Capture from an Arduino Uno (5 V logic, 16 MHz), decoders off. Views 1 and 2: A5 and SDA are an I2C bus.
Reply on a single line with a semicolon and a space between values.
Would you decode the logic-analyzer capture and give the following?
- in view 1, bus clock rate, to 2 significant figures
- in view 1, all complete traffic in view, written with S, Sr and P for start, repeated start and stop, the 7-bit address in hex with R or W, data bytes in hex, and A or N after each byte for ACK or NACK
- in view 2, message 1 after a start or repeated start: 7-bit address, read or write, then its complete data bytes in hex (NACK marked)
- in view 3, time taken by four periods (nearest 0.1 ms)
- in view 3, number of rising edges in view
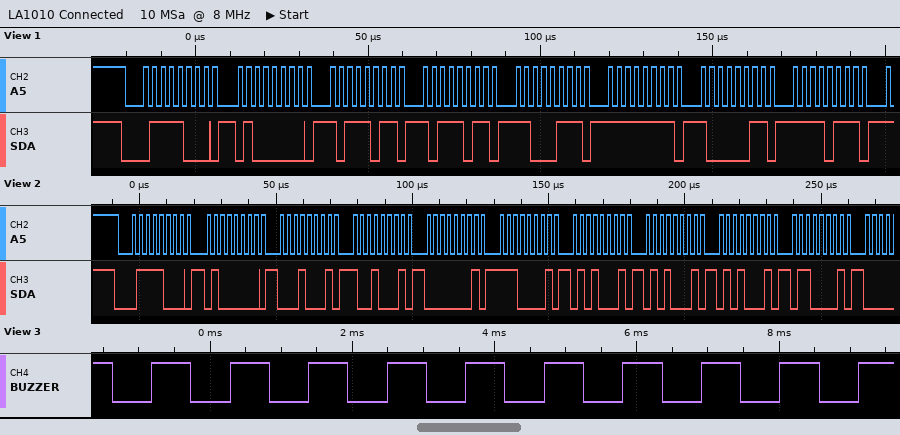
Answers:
400 kHz; S 3CW A 40 A BB A BB A C7 A FF A 83 A F7 A; 0x3C write: 40 11 91 01 E1 51 51 51 61; 4.4 ms; 10
